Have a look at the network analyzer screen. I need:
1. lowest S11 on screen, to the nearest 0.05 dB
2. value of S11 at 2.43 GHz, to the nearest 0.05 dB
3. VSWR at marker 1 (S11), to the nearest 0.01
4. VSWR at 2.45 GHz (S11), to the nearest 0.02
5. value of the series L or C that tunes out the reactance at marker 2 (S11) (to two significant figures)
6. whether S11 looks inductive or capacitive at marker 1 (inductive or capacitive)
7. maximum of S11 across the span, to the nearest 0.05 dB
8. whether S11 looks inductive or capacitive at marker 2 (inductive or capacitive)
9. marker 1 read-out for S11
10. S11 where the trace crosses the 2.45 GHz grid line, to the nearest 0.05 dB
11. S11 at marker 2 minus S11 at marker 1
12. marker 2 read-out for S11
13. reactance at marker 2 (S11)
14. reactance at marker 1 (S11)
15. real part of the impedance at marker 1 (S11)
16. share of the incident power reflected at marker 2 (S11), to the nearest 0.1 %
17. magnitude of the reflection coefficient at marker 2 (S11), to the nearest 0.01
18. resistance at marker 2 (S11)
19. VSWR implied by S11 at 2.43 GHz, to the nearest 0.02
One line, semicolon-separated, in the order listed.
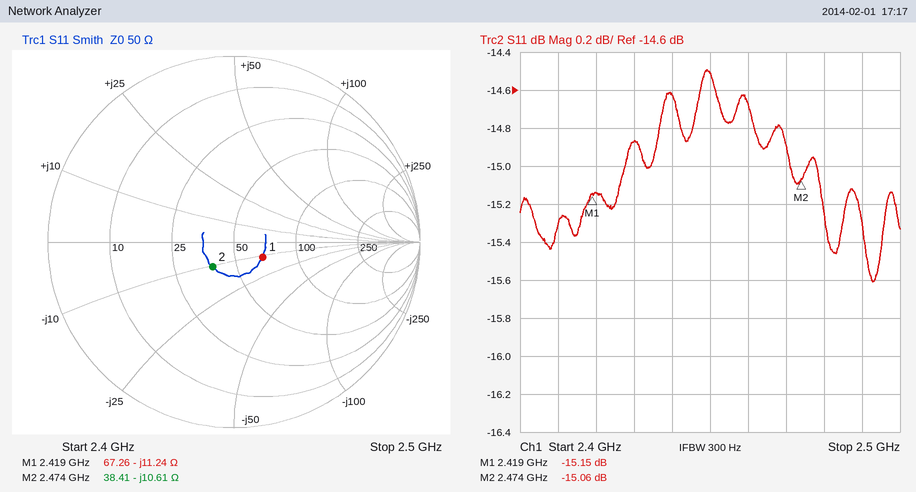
-15.60 dB; -14.85 dB; 1.42; 1.46; 680 pH; capacitive; -14.50 dB; capacitive; -15.15 dB; -14.50 dB; 0.09 dB; -15.06 dB; -10.61 Ω; -11.24 Ω; 67.26 Ω; 3.1 %; 0.18; 38.41 Ω; 1.44
